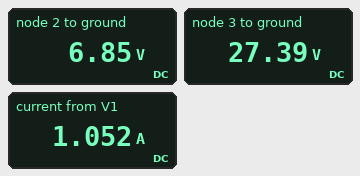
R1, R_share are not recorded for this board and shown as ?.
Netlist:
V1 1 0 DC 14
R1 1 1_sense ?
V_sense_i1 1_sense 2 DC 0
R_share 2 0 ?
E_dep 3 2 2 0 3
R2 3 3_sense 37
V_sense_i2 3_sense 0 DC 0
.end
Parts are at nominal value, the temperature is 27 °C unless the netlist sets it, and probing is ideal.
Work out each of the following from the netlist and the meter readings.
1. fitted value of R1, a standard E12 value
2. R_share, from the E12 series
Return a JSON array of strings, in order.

["6.8 Ω", "22 Ω"]
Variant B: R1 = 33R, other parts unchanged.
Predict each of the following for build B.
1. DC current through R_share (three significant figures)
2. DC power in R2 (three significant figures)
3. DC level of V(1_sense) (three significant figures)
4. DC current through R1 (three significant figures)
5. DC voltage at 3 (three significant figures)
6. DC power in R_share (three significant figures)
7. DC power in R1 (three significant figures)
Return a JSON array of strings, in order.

["105 mA", "2.30 W", "2.31 V", "354 mA", "9.23 V", "242 mW", "4.14 W"]
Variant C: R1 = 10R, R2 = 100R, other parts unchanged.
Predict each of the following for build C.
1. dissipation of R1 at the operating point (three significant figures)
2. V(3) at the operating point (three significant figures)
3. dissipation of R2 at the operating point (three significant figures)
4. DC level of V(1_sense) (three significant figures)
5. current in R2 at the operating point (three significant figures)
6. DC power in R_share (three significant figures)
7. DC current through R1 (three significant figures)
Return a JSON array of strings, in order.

["4.16 W", "30.2 V", "9.12 W", "7.55 V", "302 mA", "2.59 W", "645 mA"]
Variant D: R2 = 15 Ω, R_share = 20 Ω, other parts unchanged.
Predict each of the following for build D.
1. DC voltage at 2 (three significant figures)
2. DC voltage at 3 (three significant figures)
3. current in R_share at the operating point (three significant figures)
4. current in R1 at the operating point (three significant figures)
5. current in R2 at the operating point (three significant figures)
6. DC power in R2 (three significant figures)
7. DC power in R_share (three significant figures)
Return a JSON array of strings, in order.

["4.44 V", "17.8 V", "222 mA", "1.41 A", "1.18 A", "21.0 W", "986 mW"]
